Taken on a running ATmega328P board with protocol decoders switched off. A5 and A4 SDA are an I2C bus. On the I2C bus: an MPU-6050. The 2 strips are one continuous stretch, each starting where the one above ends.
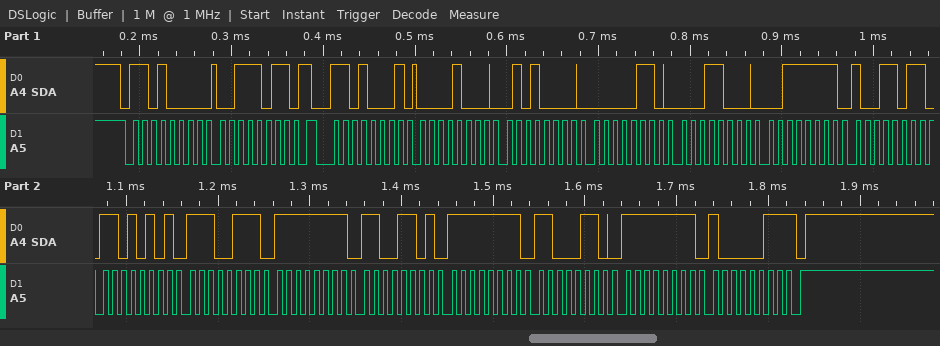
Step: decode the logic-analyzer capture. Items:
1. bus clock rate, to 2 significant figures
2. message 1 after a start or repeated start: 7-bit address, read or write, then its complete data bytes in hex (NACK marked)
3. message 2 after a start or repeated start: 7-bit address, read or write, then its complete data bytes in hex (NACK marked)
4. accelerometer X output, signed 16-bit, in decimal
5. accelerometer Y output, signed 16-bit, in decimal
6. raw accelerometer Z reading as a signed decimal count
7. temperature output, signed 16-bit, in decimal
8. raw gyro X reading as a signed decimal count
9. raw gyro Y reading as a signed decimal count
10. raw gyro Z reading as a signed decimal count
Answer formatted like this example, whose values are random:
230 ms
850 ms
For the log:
100 kHz
0x68 write: 3B
0x68 read: 08 50 06 18 3F 9B D5 E7 FF CD FF C6 FF 83 NACK
2128
1560
16283
-10777
-51
-58
-125
